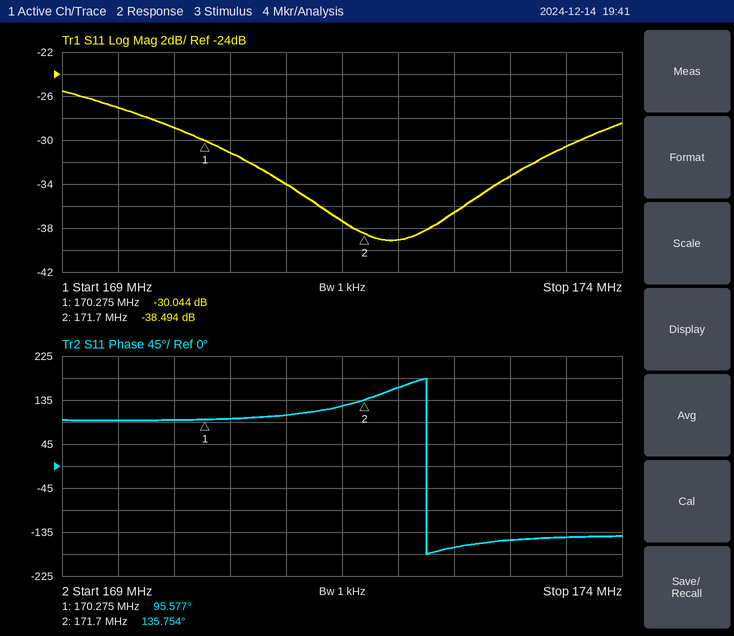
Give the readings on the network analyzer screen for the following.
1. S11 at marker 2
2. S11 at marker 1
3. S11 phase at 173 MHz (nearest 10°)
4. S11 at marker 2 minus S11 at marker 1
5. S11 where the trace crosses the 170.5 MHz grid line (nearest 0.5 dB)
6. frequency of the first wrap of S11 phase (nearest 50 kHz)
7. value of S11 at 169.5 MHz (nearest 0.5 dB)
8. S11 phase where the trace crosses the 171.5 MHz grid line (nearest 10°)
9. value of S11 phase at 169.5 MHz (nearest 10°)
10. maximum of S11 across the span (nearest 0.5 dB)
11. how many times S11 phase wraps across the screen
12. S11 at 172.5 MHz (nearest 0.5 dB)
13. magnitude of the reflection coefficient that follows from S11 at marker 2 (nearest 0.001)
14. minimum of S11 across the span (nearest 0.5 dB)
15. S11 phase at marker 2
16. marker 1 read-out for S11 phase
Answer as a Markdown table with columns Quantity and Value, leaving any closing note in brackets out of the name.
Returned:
| Quantity | Value |
|---|---|
| S11 at marker 2 | -38.494 dB |
| S11 at marker 1 | -30.044 dB |
| S11 phase at 173 MHz | -150° |
| S11 at marker 2 minus S11 at marker 1 | -8.450 dB |
| S11 where the trace crosses the 170.5 MHz grid line | -31.0 dB |
| frequency of the first wrap of S11 phase | 172.25 MHz |
| value of S11 at 169.5 MHz | -27.0 dB |
| S11 phase where the trace crosses the 171.5 MHz grid line | 120° |
| value of S11 phase at 169.5 MHz | 90° |
| maximum of S11 across the span | -25.5 dB |
| how many times S11 phase wraps across the screen | 1 |
| S11 at 172.5 MHz | -36.5 dB |
| magnitude of the reflection coefficient that follows from S11 at marker 2 | 0.012 |
| minimum of S11 across the span | -39.0 dB |
| S11 phase at marker 2 | 135.754° |
| marker 1 read-out for S11 phase | 95.577° |
